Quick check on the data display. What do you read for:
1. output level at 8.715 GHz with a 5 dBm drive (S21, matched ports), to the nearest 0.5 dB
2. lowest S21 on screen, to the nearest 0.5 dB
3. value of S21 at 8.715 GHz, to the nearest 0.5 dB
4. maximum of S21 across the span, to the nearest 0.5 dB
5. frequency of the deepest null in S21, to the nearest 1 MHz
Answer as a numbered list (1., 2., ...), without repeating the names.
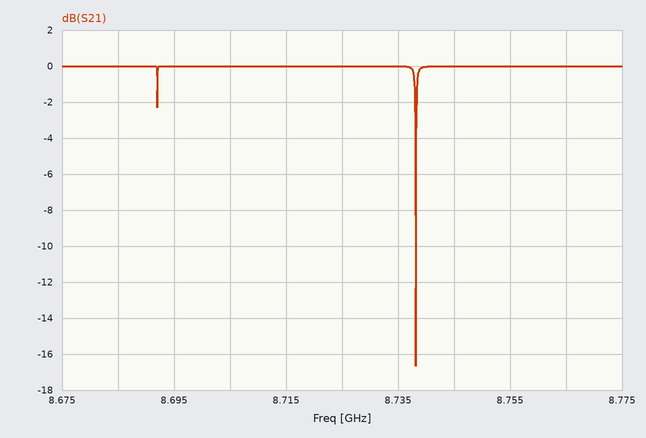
1. 5.0 dBm
2. -16.5 dB
3. 0.0 dB
4. 0.0 dB
5. 8.738 GHz
